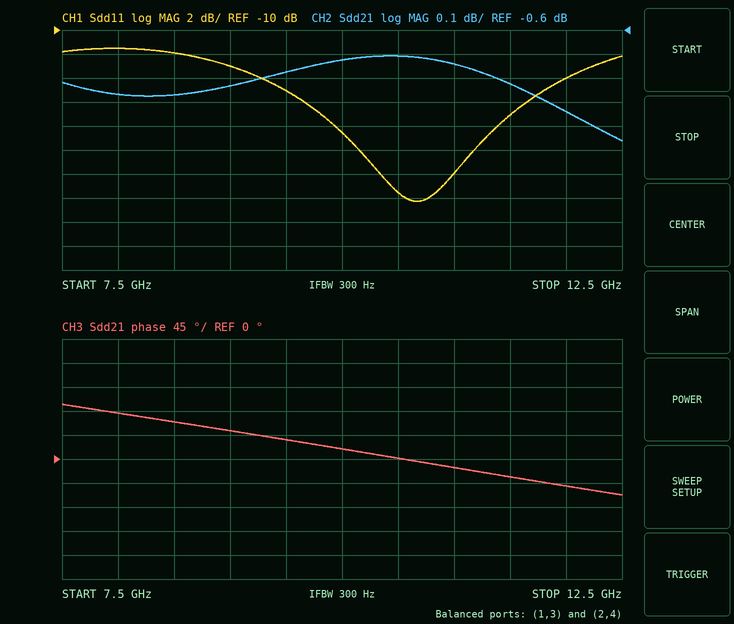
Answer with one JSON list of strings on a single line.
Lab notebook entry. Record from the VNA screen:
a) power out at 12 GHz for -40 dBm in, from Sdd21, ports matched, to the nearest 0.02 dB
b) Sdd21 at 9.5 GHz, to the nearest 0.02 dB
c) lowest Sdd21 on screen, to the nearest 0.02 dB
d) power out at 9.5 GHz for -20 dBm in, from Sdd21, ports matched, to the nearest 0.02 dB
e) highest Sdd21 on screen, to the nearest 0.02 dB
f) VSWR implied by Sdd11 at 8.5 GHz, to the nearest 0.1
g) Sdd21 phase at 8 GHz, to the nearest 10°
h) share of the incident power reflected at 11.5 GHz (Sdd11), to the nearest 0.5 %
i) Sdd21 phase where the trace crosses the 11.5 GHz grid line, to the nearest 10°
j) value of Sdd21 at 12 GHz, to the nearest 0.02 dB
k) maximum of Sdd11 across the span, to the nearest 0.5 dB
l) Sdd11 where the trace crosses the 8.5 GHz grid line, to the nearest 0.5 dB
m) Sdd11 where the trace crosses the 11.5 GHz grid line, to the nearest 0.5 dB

["-40.94 dBm", "-0.78 dB", "-1.06 dB", "-20.78 dBm", "-0.70 dB", "1.7", "90°", "2.0 %", "-30°", "-0.94 dB", "-11.5 dB", "-12.0 dB", "-17.0 dB"]
